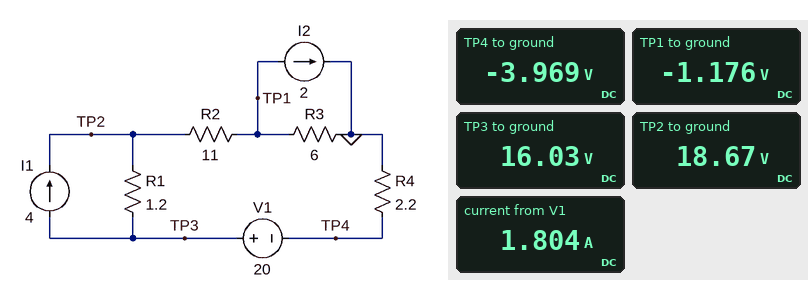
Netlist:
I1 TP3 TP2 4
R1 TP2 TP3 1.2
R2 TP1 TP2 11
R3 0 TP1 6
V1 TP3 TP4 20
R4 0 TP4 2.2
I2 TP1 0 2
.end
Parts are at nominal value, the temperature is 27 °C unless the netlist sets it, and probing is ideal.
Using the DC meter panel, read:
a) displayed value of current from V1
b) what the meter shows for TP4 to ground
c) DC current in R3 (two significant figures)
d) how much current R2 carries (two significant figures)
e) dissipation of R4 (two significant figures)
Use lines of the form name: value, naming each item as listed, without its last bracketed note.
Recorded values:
displayed value of current from V1: 1.804 A
what the meter shows for TP4 to ground: -3.969 V
DC current in R3: 200 mA
how much current R2 carries: 1.8 A
dissipation of R4: 7.2 W
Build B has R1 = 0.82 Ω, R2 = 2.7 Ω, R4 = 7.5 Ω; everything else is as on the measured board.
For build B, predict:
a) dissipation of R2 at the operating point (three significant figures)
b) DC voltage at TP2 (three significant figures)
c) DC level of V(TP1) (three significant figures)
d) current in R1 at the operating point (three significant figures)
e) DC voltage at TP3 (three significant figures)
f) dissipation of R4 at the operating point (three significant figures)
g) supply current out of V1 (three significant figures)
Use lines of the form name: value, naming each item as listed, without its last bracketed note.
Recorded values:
dissipation of R2 at the operating point: 11.6 W
DC voltage at TP2: 6.03 V
DC level of V(TP1): 437 mV
current in R1 at the operating point: 1.93 A
DC voltage at TP3: 4.45 V
dissipation of R4 at the operating point: 32.2 W
supply current out of V1: 2.07 A
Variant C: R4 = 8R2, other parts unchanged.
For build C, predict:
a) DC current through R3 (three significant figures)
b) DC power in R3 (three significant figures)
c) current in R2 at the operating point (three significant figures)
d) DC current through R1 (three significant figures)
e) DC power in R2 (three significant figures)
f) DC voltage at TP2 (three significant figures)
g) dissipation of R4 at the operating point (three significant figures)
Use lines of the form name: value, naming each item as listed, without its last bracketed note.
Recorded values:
DC current through R3: 606 mA
DC power in R3: 2.20 W
current in R2 at the operating point: 1.39 A
DC current through R1: 2.61 A
DC power in R2: 21.4 W
DC voltage at TP2: 11.7 V
dissipation of R4 at the operating point: 15.9 W
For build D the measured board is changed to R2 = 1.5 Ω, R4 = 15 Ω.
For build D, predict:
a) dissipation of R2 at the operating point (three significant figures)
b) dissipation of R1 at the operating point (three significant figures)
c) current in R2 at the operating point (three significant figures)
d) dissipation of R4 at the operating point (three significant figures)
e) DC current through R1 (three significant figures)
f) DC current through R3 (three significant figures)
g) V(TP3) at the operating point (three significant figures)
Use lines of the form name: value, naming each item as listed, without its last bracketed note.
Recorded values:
dissipation of R2 at the operating point: 3.62 W
dissipation of R1 at the operating point: 7.19 W
current in R2 at the operating point: 1.55 A
dissipation of R4 at the operating point: 36.2 W
DC current through R1: 2.45 A
DC current through R3: 447 mA
V(TP3) at the operating point: -3.29 V
